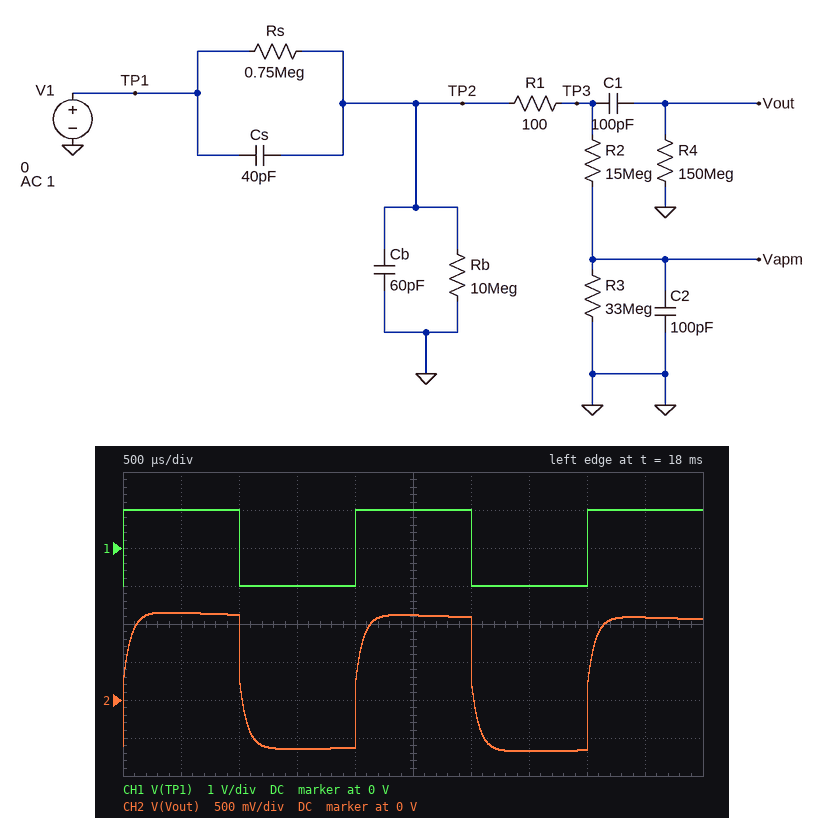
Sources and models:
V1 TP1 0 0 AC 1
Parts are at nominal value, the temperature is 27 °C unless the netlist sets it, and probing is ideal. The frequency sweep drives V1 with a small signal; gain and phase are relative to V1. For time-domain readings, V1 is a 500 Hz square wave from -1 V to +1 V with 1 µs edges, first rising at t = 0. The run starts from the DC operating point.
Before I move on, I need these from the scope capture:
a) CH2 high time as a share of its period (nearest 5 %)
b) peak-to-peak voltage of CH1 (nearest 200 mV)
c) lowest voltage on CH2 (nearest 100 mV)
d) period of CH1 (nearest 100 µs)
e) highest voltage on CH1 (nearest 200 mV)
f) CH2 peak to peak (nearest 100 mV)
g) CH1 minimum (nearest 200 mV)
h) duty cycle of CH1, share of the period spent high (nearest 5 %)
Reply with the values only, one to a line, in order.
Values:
50 %
2.0 V
-700 mV
2.0 ms
1.0 V
1.8 V
-1.0 V
50 %
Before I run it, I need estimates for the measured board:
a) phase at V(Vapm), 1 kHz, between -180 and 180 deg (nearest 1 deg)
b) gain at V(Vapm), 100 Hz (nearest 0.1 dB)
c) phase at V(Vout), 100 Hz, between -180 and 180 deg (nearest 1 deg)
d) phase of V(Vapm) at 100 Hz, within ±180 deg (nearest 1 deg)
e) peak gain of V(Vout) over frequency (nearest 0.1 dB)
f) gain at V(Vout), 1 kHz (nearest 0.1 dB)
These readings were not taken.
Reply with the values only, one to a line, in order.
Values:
-93 deg
-5.7 dB
4 deg
-35 deg
-0.9 dB
-1.6 dB
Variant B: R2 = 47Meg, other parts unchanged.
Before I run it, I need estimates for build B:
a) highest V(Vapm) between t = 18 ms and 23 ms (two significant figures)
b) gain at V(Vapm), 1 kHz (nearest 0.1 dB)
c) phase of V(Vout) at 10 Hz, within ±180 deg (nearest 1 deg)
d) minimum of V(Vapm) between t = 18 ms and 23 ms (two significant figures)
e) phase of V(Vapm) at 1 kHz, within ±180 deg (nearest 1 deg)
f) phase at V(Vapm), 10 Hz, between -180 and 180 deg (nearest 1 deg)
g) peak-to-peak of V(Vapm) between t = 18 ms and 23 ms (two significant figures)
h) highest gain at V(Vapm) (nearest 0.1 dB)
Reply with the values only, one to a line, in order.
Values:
89 mV
-30.8 dB
46 deg
-90 mV
-98 deg
-7 deg
180 mV
-8.4 dB
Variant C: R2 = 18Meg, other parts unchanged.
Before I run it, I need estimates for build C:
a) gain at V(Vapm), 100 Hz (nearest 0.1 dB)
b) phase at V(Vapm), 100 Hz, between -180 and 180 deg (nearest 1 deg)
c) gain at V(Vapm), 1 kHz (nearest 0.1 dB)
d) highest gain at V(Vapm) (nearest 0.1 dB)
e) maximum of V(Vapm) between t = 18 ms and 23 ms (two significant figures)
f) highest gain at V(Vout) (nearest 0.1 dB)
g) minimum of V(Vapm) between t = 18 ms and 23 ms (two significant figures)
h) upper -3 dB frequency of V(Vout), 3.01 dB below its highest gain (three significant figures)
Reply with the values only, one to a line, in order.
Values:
-6.5 dB
-38 deg
-22.7 dB
-4.5 dB
220 mV
-0.9 dB
-220 mV
3.00 kHz
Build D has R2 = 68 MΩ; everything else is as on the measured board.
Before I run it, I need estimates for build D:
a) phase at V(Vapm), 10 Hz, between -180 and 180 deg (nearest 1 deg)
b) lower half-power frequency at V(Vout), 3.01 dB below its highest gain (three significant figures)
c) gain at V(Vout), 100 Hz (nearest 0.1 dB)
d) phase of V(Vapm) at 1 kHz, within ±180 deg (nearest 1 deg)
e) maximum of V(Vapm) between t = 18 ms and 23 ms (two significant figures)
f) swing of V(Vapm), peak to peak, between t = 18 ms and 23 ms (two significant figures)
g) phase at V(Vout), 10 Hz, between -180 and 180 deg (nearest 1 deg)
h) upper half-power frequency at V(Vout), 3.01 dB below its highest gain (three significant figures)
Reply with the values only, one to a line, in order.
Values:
-8 deg
10.4 Hz
-0.8 dB
-99 deg
62 mV
120 mV
46 deg
2.97 kHz
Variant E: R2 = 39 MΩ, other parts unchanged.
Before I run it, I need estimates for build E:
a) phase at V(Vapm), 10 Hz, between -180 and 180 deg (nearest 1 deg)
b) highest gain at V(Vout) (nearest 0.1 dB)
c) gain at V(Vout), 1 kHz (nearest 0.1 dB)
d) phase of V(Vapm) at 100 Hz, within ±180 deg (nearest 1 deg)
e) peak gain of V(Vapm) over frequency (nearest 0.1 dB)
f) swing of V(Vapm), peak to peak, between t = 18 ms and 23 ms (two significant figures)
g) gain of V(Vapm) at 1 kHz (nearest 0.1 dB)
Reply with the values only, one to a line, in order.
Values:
-7 deg
-0.8 dB
-1.4 dB
-50 deg
-7.5 dB
210 mV
-29.2 dB
